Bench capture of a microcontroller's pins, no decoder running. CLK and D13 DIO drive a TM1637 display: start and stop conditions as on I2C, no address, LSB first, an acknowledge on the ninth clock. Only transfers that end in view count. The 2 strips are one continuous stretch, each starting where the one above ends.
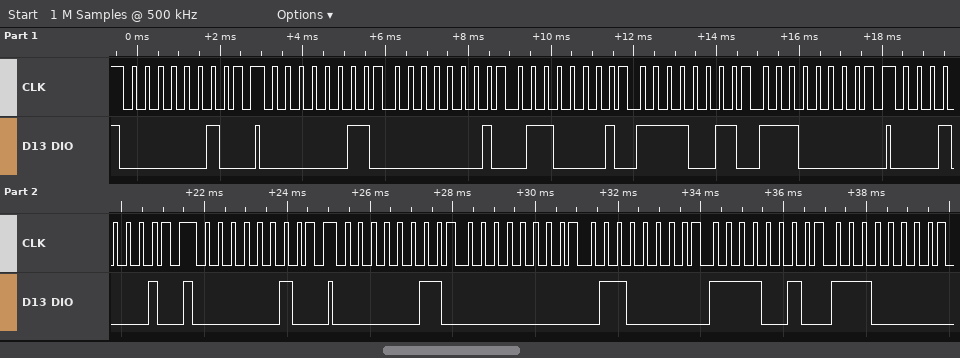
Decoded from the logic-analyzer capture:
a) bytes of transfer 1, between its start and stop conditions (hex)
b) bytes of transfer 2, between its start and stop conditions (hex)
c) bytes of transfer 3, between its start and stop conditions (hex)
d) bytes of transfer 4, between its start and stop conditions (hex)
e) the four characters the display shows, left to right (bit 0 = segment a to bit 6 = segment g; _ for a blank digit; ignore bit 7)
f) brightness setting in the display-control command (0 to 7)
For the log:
40
C0 80 86 CF 07
88
40
_137
0
